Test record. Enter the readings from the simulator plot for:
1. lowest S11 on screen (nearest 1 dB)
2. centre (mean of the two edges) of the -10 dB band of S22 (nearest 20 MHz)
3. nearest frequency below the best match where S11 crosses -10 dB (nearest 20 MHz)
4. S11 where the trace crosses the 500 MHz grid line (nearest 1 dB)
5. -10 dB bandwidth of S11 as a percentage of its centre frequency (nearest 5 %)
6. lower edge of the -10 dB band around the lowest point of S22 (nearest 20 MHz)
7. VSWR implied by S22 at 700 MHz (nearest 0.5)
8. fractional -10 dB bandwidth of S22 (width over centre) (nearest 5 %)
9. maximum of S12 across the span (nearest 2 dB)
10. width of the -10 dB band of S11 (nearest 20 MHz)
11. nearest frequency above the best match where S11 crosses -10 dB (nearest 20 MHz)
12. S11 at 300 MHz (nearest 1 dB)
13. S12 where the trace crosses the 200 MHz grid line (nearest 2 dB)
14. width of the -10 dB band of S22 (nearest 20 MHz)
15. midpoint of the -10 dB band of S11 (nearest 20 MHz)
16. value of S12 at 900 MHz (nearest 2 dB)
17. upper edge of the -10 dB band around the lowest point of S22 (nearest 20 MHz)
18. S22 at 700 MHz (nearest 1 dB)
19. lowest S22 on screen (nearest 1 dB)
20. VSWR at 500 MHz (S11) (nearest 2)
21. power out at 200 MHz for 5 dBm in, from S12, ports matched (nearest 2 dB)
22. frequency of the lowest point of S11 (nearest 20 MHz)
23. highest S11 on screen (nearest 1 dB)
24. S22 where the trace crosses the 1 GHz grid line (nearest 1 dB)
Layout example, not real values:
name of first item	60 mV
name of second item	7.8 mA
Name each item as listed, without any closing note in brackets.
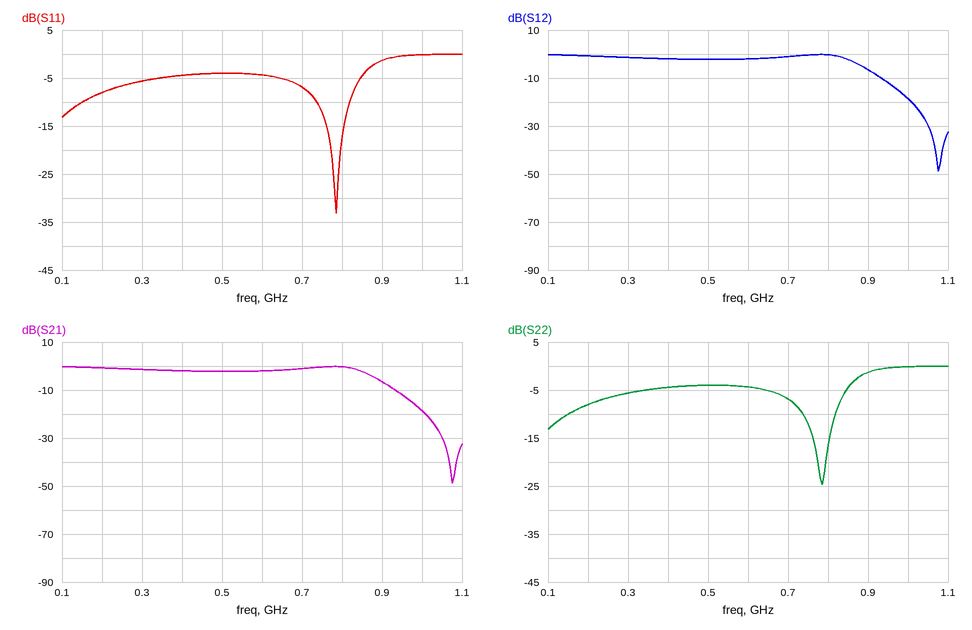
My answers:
lowest S11 on screen	-33 dB
centre (mean of the two edges) of the -10 dB band of S22	780 MHz
nearest frequency below the best match where S11 crosses -10 dB	740 MHz
S11 where the trace crosses the 500 MHz grid line	-4 dB
-10 dB bandwidth of S11 as a percentage of its centre frequency	10 %
lower edge of the -10 dB band around the lowest point of S22	740 MHz
VSWR implied by S22 at 700 MHz	2.5
fractional -10 dB bandwidth of S22 (width over centre)	10 %
maximum of S12 across the span	0 dB
width of the -10 dB band of S11	80 MHz
nearest frequency above the best match where S11 crosses -10 dB	820 MHz
S11 at 300 MHz	-6 dB
S12 where the trace crosses the 200 MHz grid line	0 dB
width of the -10 dB band of S22	80 MHz
midpoint of the -10 dB band of S11	780 MHz
value of S12 at 900 MHz	-6 dB
upper edge of the -10 dB band around the lowest point of S22	820 MHz
S22 at 700 MHz	-7 dB
lowest S22 on screen	-25 dB
VSWR at 500 MHz (S11)	4
power out at 200 MHz for 5 dBm in, from S12, ports matched	4 dBm
frequency of the lowest point of S11	780 MHz
highest S11 on screen	0 dB
S22 where the trace crosses the 1 GHz grid line	0 dB
